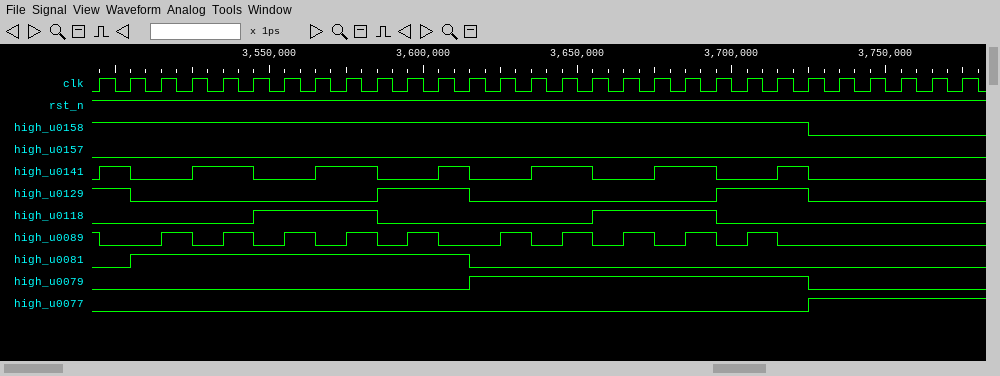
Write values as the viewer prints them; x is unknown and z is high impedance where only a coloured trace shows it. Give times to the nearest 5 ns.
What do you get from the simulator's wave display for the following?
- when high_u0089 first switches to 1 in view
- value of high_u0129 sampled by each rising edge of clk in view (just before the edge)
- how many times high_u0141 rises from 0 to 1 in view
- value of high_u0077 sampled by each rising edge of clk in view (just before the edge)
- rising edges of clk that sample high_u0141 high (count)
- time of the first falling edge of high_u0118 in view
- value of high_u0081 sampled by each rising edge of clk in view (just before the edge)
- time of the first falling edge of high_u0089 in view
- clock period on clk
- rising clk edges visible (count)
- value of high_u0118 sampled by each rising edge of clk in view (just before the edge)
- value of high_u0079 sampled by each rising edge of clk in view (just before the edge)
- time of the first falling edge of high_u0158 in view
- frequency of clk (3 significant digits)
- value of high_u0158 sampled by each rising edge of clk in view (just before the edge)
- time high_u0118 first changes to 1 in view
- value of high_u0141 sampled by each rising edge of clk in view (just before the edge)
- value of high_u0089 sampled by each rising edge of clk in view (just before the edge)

3515 ns
1 1 0 0 0 0 0 0 0 0 1 1 1 0 0 0 0 0 0 0 0 1 1 1 0 0 0 0 0
7
0 0 0 0 0 0 0 0 0 0 0 0 0 0 0 0 0 0 0 0 0 0 0 0 1 1 1 1 1
11
3585 ns
0 0 1 1 1 1 1 1 1 1 1 1 1 0 0 0 0 0 0 0 0 0 0 0 0 0 0 0 0
3495 ns
10 ns
29
0 0 0 0 0 0 1 1 1 1 0 0 0 0 0 0 0 1 1 1 1 0 0 0 0 0 0 0 0
0 0 0 0 0 0 0 0 0 0 0 0 0 1 1 1 1 1 1 1 1 1 1 1 0 0 0 0 0
3725 ns
100 MHz
1 1 1 1 1 1 1 1 1 1 1 1 1 1 1 1 1 1 1 1 1 1 1 1 0 0 0 0 0
3545 ns
0 1 0 0 1 1 0 0 1 1 0 0 1 0 0 1 1 0 0 1 1 0 0 1 0 0 0 0 0
1 0 0 1 0 1 0 1 0 1 0 1 0 0 1 0 1 0 1 0 1 0 1 0 0 0 0 0 0
